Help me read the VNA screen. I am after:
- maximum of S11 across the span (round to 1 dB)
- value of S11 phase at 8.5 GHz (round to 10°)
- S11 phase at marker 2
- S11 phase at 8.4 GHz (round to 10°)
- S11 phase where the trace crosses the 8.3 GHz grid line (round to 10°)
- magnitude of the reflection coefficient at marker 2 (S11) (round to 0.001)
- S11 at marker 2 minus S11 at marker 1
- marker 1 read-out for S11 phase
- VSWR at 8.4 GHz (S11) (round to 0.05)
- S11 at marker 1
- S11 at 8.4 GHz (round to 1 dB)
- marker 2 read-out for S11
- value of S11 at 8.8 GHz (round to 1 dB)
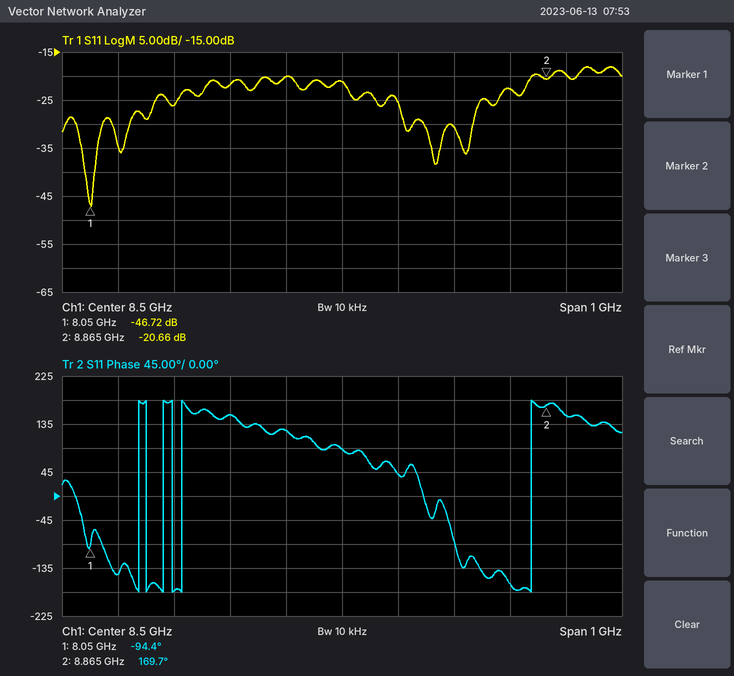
-18 dB
90°
169.7°
120°
150°
0.093
26.06 dB
-94.4°
1.20
-46.72 dB
-20 dB
-20.66 dB
-23 dB
